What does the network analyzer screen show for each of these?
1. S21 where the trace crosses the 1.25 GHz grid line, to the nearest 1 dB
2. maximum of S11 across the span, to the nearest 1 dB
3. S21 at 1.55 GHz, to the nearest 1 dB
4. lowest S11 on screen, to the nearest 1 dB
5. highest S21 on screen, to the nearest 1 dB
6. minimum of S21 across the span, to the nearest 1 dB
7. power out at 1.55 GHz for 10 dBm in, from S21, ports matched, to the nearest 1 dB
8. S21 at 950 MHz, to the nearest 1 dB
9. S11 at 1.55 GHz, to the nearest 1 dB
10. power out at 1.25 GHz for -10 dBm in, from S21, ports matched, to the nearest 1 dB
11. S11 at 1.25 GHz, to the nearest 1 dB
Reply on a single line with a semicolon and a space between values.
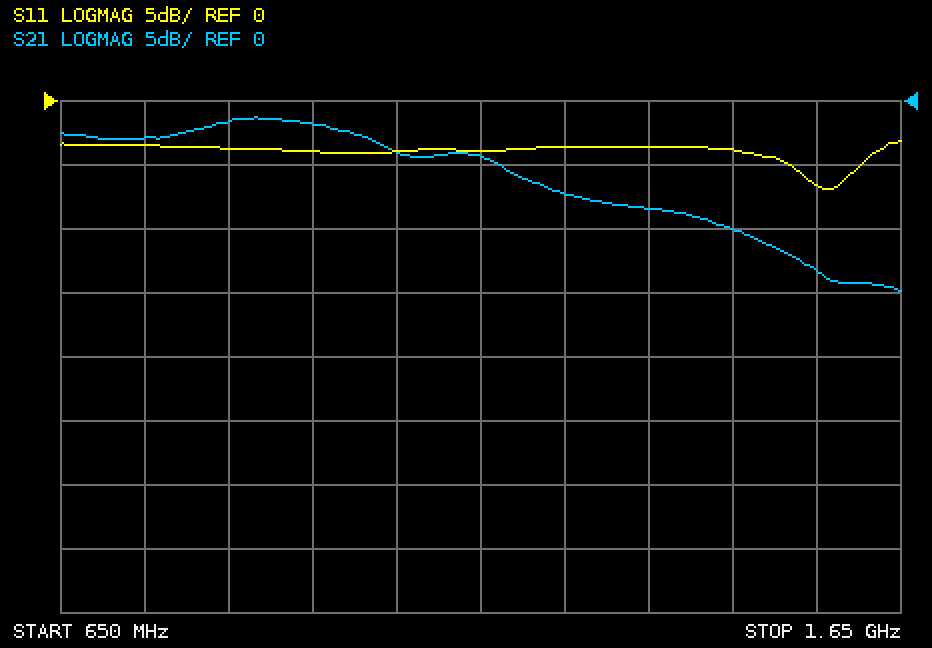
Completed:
-7 dB; -3 dB; -13 dB; -7 dB; -1 dB; -15 dB; -3 dBm; -2 dB; -7 dB; -17 dBm; -4 dB
